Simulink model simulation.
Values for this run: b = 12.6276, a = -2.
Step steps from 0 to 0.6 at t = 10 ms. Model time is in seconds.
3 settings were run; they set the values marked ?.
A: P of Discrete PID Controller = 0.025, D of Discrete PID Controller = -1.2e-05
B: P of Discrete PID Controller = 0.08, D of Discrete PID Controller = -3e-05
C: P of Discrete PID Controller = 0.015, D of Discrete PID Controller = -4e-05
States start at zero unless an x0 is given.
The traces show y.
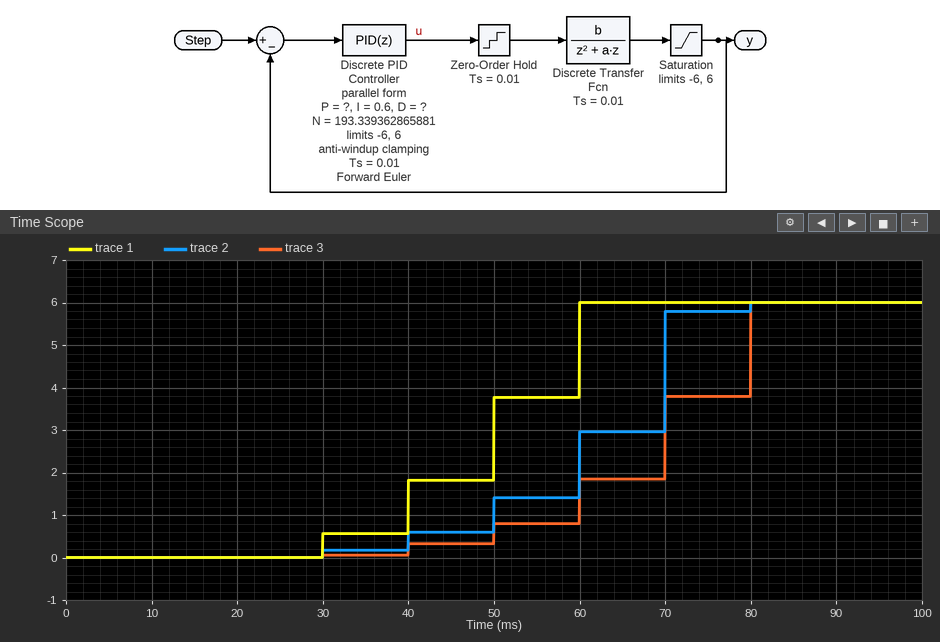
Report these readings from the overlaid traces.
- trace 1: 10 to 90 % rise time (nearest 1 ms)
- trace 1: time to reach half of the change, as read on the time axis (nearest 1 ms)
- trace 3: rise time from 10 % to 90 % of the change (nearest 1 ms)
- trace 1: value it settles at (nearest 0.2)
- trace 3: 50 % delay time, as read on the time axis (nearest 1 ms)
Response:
20 ms
50 ms
30 ms
6.0
70 ms
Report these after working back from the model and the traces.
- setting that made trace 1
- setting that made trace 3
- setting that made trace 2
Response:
B
C
A
